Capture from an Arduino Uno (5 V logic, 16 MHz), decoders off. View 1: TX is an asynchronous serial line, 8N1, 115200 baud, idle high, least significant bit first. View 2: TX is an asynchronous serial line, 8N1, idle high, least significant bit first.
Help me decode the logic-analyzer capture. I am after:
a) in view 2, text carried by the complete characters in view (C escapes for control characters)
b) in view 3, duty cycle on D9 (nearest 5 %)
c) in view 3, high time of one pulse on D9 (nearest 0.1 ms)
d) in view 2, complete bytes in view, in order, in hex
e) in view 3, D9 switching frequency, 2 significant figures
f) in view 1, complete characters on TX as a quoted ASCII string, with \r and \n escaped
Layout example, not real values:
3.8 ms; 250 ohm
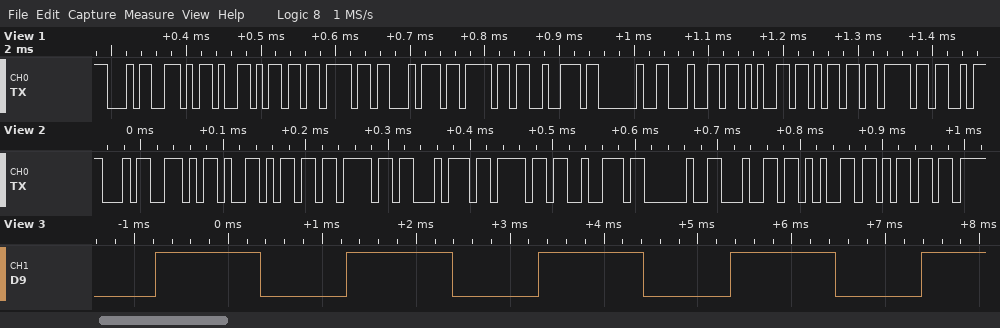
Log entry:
"4-motor dem"; 55 %; 1.1 ms; 0x34 0x2D 0x6D 0x6F 0x74 0x6F 0x72 0x20 0x64 0x65 0x6D; 490 Hz; "4-motor demo"
